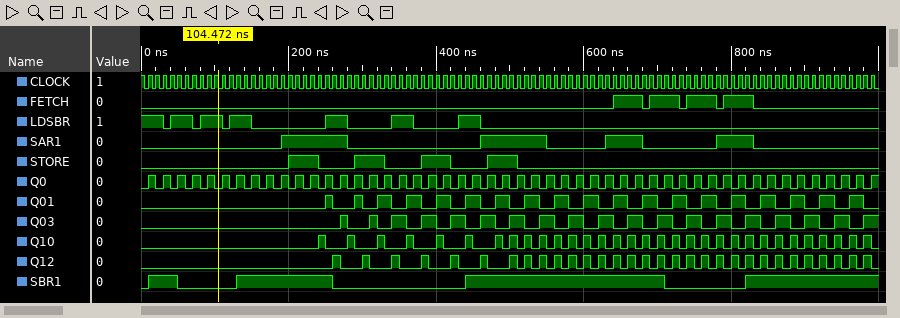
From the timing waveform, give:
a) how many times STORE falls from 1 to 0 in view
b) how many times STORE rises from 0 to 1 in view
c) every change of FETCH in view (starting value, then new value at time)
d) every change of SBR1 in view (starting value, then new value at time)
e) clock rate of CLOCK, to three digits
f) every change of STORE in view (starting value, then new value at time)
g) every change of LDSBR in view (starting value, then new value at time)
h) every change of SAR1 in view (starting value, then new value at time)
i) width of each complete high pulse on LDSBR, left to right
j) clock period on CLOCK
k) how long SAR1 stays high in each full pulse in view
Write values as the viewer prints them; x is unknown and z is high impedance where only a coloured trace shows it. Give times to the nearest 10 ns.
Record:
4
4
0, 1 at 640 ns, 0 at 680 ns, 1 at 690 ns, 0 at 730 ns, 1 at 740 ns, 0 at 780 ns, 1 at 790 ns, 0 at 830 ns
0, 1 at 10 ns, 0 at 50 ns, 1 at 130 ns, 0 at 260 ns, 1 at 440 ns, 0 at 710 ns, 1 at 820 ns
100 MHz
0, 1 at 200 ns, 0 at 240 ns, 1 at 290 ns, 0 at 330 ns, 1 at 380 ns, 0 at 420 ns, 1 at 470 ns, 0 at 510 ns
1, 0 at 30 ns, 1 at 40 ns, 0 at 70 ns, 1 at 80 ns, 0 at 110 ns, 1 at 120 ns, 0 at 150 ns, 1 at 250 ns, 0 at 280 ns, 1 at 340 ns, 0 at 370 ns, 1 at 430 ns, 0 at 460 ns
0, 1 at 190 ns, 0 at 280 ns, 1 at 460 ns, 0 at 550 ns, 1 at 630 ns, 0 at 680 ns, 1 at 780 ns, 0 at 830 ns
30 ns, 30 ns, 30 ns, 30 ns, 30 ns, 30 ns
10 ns
90 ns, 90 ns, 50 ns, 50 ns
